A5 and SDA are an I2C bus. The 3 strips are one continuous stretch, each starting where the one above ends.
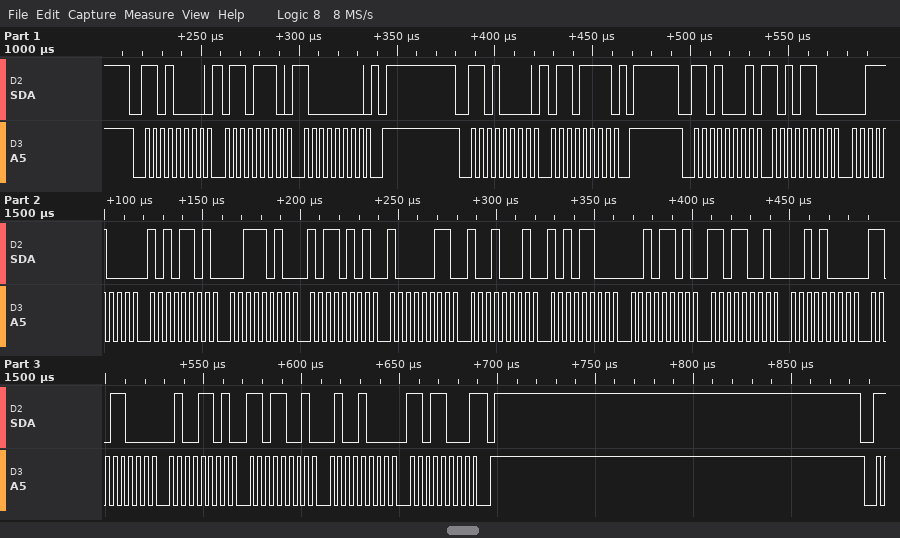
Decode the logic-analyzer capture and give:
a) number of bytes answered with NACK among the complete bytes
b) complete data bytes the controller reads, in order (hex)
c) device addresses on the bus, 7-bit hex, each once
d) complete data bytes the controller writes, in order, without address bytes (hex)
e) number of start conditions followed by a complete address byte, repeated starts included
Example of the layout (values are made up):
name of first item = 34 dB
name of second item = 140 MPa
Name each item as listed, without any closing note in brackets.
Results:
number of bytes answered with NACK among the complete bytes = 1
complete data bytes the controller reads, in order = AC 38 AD 3A B5 83 91 AC 2D D9 28 D8 4D D9 48 D8
device addresses on the bus, 7-bit hex, each once = 0x68
complete data bytes the controller writes, in order, without address bytes = 6E 80 6F
number of start conditions followed by a complete address byte, repeated starts included = 3
